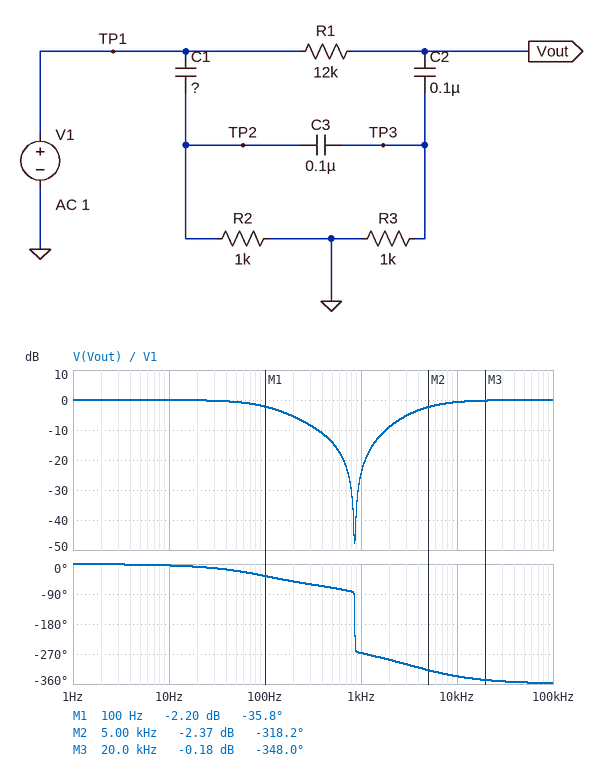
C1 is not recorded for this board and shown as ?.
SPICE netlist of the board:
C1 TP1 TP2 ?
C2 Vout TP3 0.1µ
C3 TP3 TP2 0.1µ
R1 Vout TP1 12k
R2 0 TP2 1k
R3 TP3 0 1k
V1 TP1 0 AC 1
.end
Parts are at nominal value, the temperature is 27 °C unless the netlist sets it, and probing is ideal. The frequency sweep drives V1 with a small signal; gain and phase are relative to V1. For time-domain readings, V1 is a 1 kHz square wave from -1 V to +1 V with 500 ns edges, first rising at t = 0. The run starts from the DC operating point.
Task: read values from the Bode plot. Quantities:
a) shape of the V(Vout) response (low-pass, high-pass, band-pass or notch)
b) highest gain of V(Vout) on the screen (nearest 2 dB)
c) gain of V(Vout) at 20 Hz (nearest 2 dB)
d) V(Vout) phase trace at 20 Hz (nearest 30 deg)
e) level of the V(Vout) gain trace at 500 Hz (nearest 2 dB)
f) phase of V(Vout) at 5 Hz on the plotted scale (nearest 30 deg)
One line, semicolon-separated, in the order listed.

notch; 0 dB; 0 dB; 0 deg; -14 dB; 0 deg
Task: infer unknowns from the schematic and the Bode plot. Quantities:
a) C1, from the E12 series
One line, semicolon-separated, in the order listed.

120 nF
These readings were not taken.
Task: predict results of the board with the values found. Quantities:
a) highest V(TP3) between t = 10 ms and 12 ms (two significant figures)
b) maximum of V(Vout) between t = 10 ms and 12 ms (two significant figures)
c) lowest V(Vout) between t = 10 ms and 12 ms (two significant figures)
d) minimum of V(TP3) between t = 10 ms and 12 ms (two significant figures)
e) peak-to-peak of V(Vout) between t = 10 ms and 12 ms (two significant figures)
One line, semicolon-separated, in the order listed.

2.0 V; 1.8 V; -1.8 V; -2.0 V; 3.6 V
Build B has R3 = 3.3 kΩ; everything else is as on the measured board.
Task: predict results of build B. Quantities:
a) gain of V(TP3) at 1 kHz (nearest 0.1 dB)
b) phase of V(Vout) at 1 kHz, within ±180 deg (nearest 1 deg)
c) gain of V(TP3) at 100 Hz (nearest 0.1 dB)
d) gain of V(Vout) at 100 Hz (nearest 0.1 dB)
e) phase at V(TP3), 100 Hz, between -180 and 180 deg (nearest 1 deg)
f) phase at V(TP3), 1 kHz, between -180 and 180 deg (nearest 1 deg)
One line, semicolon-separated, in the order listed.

-8.8 dB; 64 deg; -17.3 dB; -2.5 dB; 41 deg; 68 deg
